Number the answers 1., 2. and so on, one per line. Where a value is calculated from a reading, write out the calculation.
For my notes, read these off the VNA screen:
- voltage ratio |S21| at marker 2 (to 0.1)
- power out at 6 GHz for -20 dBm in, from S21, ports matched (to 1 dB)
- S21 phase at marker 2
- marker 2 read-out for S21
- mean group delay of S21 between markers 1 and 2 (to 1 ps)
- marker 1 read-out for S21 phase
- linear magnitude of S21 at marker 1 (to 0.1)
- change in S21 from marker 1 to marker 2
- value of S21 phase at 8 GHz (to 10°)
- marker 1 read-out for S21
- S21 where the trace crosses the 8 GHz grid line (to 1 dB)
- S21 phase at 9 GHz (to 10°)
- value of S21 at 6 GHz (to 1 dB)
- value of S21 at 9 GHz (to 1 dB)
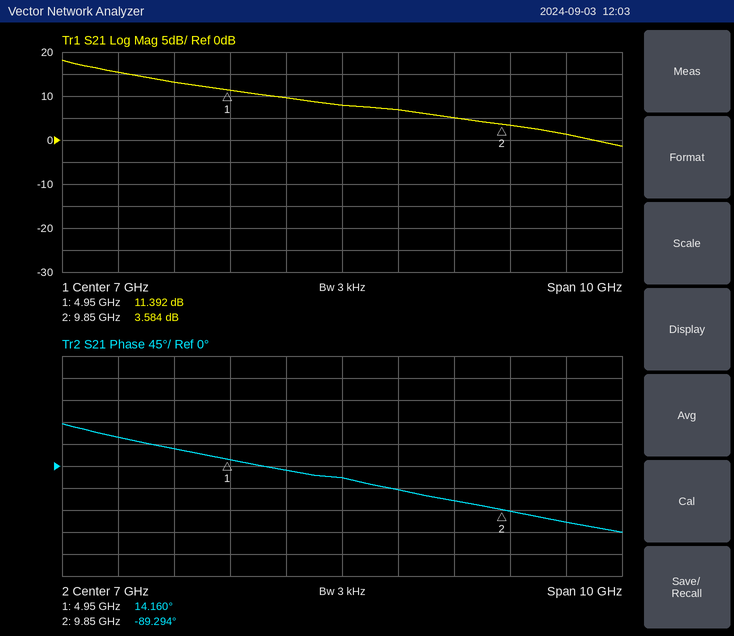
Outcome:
1. 10^(3.584/20) ≈ 1.5
2. -20 dBm + (10 dB) = -10 dBm
3. -89.294°
4. 3.584 dB
5. −(-89.294° − (14.16°))/(360° × 4.9 GHz) ≈ 59 ps
6. 14.160°
7. 10^(11.392/20) ≈ 3.7
8. 3.584 − (11.392) = -7.808 dB
9. -50°
10. 11.392 dB
11. 7 dB
12. -70°
13. 10 dB
14. 5 dB
